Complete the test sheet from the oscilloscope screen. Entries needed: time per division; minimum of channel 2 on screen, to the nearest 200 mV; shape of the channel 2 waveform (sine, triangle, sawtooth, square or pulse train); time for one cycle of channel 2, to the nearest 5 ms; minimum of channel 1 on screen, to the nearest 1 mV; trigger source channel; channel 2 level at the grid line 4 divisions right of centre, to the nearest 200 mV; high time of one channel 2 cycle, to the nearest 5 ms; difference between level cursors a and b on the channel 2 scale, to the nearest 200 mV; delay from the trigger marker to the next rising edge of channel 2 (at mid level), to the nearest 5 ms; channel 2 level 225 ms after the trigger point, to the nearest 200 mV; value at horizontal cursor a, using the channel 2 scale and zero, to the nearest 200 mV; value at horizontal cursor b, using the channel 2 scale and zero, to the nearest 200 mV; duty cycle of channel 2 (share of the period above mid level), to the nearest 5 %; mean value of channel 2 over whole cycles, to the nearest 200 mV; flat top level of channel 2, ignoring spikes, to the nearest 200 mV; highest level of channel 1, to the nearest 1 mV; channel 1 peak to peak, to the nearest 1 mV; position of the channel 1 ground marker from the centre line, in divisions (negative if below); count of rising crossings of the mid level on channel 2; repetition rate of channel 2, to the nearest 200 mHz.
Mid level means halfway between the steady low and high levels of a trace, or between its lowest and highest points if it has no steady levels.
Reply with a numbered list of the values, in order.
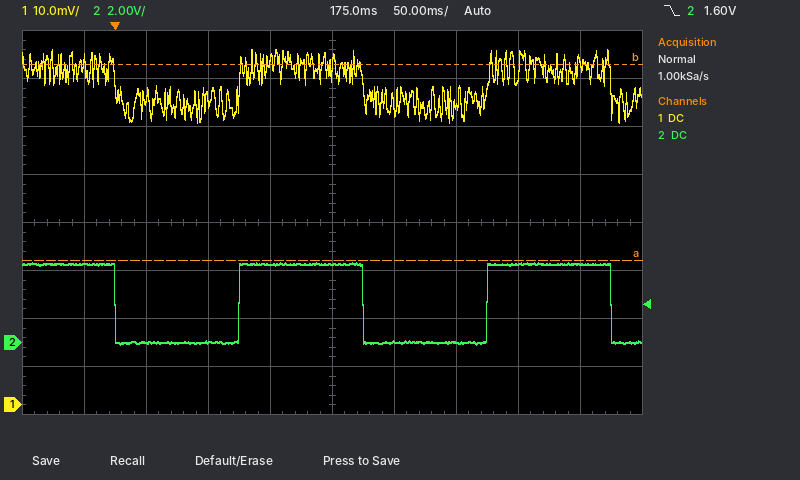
1. 50 ms
2. 0.0 V
3. square
4. 200 ms
5. 59 mV
6. channel 2
7. 3.2 V
8. 100 ms
9. 8.2 V
10. 100 ms
11. 0.0 V
12. 3.4 V
13. 11.6 V
14. 50 %
15. 1.6 V
16. 3.2 V
17. 74 mV
18. 15 mV
19. -3.8 div
20. 2
21. 5.0 Hz
